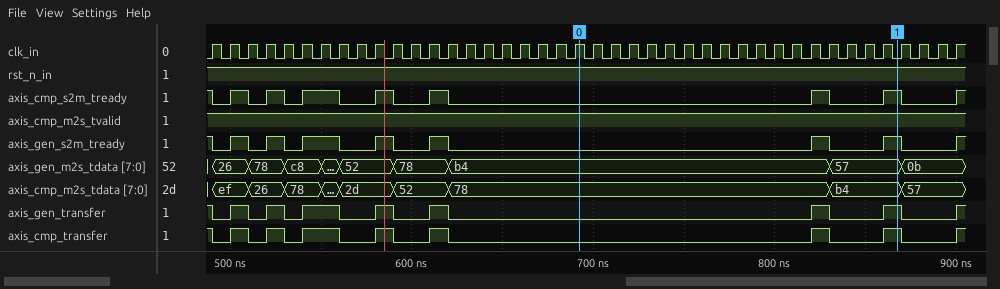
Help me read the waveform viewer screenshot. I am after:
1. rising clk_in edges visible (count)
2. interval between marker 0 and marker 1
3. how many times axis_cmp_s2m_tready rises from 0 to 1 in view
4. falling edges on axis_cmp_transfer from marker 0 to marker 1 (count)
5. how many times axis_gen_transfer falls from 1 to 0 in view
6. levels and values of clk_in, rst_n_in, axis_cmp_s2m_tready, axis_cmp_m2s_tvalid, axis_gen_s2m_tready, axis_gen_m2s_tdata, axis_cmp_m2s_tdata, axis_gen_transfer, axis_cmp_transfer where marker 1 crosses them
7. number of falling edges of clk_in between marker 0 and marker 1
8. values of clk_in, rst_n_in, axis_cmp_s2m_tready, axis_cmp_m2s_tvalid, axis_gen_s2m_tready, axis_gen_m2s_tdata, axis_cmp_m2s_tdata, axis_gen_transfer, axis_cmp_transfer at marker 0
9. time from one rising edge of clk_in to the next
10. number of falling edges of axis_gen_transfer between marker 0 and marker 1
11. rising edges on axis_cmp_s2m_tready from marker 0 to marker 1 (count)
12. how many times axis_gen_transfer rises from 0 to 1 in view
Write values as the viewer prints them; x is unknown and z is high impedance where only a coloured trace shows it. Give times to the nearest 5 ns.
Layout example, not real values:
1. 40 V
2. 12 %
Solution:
1. 42
2. 175 ns
3. 8
4. 1
5. 8
6. clk_in=0, rst_n_in=1, axis_cmp_s2m_tready=1, axis_cmp_m2s_tvalid=1, axis_gen_s2m_tready=1, axis_gen_m2s_tdata=57, axis_cmp_m2s_tdata=b4, axis_gen_transfer=1, axis_cmp_transfer=1
7. 18
8. clk_in=1, rst_n_in=1, axis_cmp_s2m_tready=0, axis_cmp_m2s_tvalid=1, axis_gen_s2m_tready=0, axis_gen_m2s_tdata=b4, axis_cmp_m2s_tdata=78, axis_gen_transfer=0, axis_cmp_transfer=0
9. 10 ns
10. 1
11. 2
12. 8
